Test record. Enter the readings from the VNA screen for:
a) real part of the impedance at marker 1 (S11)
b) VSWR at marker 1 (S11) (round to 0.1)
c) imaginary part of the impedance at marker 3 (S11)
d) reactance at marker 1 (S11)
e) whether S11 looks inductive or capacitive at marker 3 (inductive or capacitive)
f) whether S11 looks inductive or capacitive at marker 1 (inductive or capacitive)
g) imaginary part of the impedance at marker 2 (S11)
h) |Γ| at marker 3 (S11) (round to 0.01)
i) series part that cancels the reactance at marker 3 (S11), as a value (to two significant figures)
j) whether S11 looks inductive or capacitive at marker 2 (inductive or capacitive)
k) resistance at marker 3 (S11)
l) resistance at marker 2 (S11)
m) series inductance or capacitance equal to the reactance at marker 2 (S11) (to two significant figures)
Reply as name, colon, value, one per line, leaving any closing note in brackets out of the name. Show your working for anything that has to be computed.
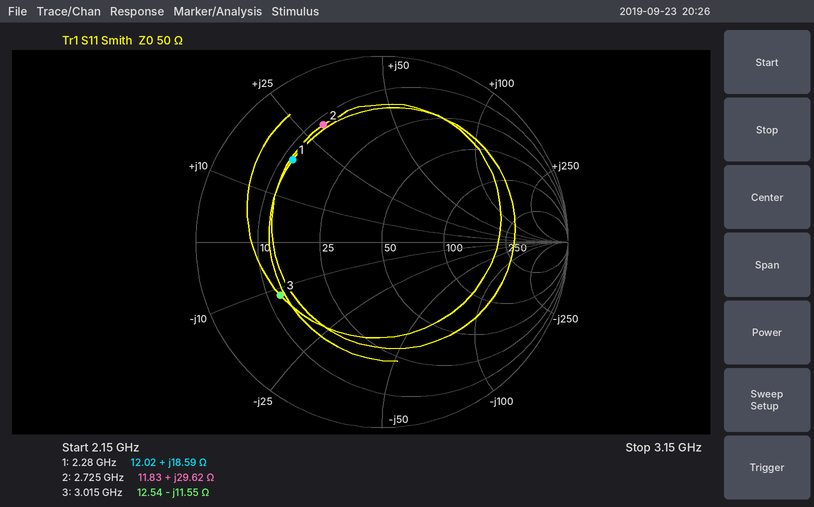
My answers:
real part of the impedance at marker 1: 12.02 Ω
VSWR at marker 1 (S11): 4.8
imaginary part of the impedance at marker 3: -11.55 Ω
reactance at marker 1: +18.59 Ω
whether S11 looks inductive or capacitive at marker 3: capacitive
whether S11 looks inductive or capacitive at marker 1: inductive
imaginary part of the impedance at marker 2: +29.62 Ω
|Γ| at marker 3 (S11): 0.62
series part that cancels the reactance at marker 3 (S11), as a value: L = 11.55 Ω/(2π × 3.015 GHz) ≈ 610 pH
whether S11 looks inductive or capacitive at marker 2: inductive
resistance at marker 3: 12.54 Ω
resistance at marker 2: 11.83 Ω
series inductance or capacitance equal to the reactance at marker 2 (S11): L = 29.62 Ω/(2π × 2.725 GHz) ≈ 1.7 nH
